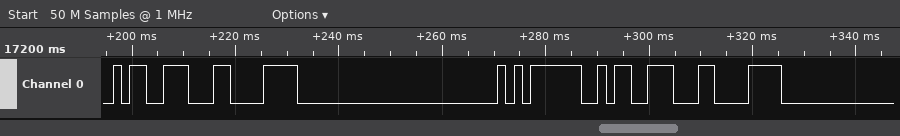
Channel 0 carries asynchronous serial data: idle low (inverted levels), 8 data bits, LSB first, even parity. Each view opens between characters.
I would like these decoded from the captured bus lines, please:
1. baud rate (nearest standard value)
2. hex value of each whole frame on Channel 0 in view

600 baud
19, 1E, 05, 19, 1E
